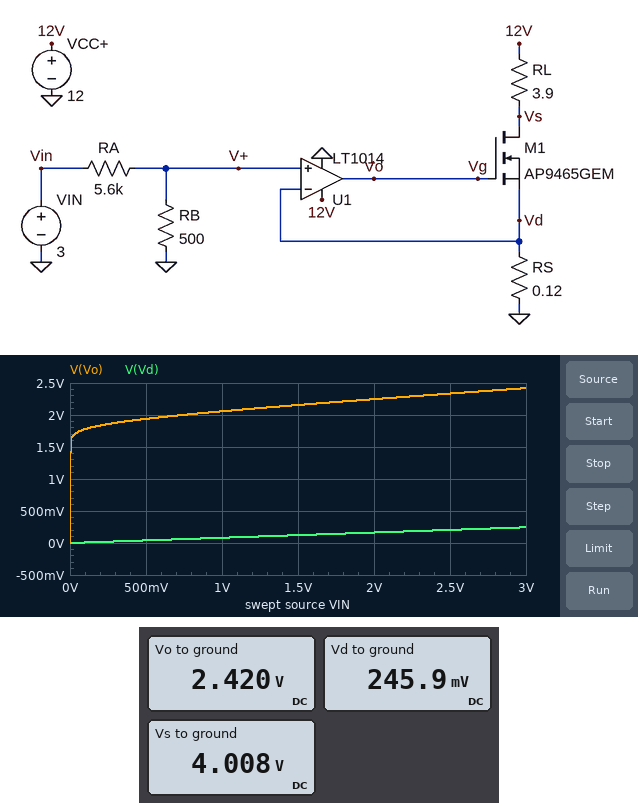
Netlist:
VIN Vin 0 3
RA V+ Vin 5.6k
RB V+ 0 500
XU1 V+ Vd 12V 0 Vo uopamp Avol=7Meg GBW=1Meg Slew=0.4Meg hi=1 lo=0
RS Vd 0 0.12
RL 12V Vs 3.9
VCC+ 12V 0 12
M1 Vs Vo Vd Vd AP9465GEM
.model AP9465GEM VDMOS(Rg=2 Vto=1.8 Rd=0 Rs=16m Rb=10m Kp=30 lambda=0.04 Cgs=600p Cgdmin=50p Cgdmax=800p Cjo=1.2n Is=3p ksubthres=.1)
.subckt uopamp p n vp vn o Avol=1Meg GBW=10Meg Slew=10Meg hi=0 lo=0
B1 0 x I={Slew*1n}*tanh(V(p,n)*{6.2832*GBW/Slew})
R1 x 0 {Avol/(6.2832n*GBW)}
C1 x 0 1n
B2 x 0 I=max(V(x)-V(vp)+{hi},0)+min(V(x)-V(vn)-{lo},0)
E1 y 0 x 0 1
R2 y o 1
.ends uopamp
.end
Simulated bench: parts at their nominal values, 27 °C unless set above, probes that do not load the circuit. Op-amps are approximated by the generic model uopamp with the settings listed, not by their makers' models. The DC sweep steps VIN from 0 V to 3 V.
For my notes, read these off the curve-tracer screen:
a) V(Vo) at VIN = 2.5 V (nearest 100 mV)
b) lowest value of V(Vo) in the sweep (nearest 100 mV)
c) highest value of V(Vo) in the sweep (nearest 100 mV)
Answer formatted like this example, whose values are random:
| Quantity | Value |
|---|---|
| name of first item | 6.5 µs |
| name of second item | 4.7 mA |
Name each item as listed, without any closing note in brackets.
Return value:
| Quantity | Value |
|---|---|
| V(Vo) at VIN = 2.5 V | 2.3 V |
| lowest value of V(Vo) in the sweep | 0 V |
| highest value of V(Vo) in the sweep | 2.4 V |
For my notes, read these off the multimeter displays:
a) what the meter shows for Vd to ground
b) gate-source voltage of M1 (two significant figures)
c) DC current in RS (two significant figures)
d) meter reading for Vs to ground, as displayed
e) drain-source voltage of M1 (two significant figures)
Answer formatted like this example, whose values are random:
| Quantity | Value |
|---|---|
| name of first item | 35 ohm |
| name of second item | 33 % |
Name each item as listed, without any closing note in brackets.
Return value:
| Quantity | Value |
|---|---|
| what the meter shows for Vd to ground | 245.9 mV |
| gate-source voltage of M1 | 2.2 V |
| DC current in RS | 2.0 A |
| meter reading for Vs to ground, as displayed | 4.008 V |
| drain-source voltage of M1 | 3.8 V |
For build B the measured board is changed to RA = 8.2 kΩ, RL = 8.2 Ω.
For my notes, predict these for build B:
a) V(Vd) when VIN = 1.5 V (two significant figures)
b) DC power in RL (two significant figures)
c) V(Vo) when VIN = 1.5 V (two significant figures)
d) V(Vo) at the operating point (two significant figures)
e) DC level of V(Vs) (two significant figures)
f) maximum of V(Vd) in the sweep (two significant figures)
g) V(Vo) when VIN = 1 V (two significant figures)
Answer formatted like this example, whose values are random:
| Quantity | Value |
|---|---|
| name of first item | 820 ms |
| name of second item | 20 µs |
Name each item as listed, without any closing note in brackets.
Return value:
| Quantity | Value |
|---|---|
| V(Vd) when VIN = 1.5 V | 86 mV |
| DC power in RL | 17 W |
| V(Vo) when VIN = 1.5 V | 2.1 V |
| V(Vo) at the operating point | 4.1 V |
| DC level of V(Vs) | 220 mV |
| maximum of V(Vd) in the sweep | 170 mV |
| V(Vo) when VIN = 1 V | 2.0 V |
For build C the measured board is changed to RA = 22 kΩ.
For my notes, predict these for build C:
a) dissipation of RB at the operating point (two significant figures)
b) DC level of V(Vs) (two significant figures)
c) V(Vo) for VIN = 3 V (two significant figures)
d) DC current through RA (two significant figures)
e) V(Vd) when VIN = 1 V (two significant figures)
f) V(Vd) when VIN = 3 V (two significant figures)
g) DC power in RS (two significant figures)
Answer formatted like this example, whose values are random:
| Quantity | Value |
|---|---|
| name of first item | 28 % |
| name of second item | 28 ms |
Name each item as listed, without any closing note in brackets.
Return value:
| Quantity | Value |
|---|---|
| dissipation of RB at the operating point | 8.9 µW |
| DC level of V(Vs) | 9.8 V |
| V(Vo) for VIN = 3 V | 2.0 V |
| DC current through RA | 130 µA |
| V(Vd) when VIN = 1 V | 22 mV |
| V(Vd) when VIN = 3 V | 67 mV |
| DC power in RS | 37 mW |
